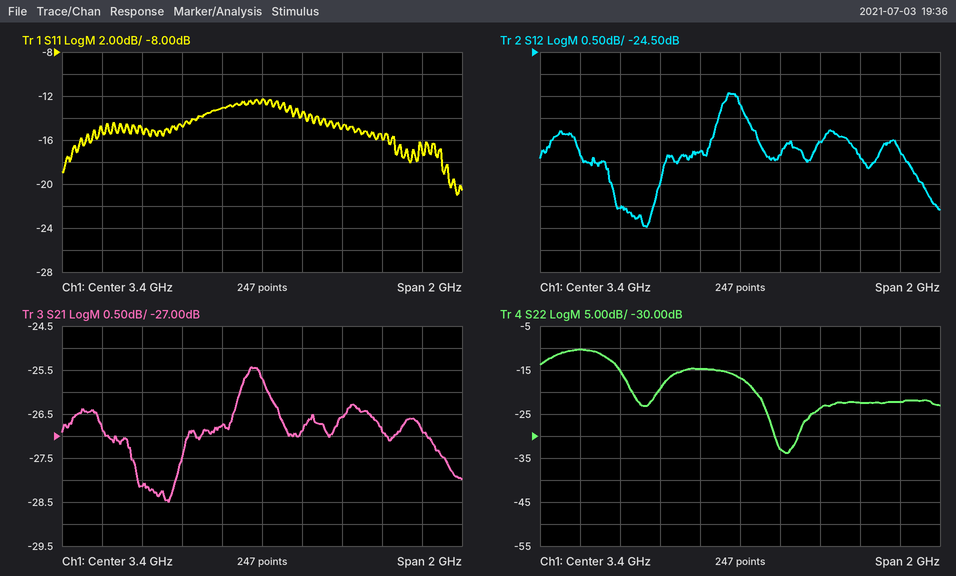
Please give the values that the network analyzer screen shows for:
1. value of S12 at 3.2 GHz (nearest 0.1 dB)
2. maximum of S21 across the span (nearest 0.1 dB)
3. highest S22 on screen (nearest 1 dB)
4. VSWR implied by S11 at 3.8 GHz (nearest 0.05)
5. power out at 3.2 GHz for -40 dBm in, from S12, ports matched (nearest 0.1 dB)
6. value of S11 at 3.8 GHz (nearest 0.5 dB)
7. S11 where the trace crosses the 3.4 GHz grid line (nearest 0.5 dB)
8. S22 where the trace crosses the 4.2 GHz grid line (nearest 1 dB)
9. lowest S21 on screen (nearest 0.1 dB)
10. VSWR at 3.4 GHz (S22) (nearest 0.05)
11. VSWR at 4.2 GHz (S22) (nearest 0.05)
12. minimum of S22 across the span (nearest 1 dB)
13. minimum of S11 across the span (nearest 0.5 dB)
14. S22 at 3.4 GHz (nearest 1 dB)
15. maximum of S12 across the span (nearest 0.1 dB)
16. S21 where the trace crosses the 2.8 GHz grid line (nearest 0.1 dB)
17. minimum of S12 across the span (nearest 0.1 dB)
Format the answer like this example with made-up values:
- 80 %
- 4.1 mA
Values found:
- -26.8 dB
- -25.4 dB
- -10 dB
- 1.45
- -66.8 dBm
- -15.0 dB
- -12.5 dB
- -22 dB
- -28.5 dB
- 1.35
- 1.15
- -34 dB
- -21.0 dB
- -17 dB
- -25.4 dB
- -28.1 dB
- -28.5 dB
